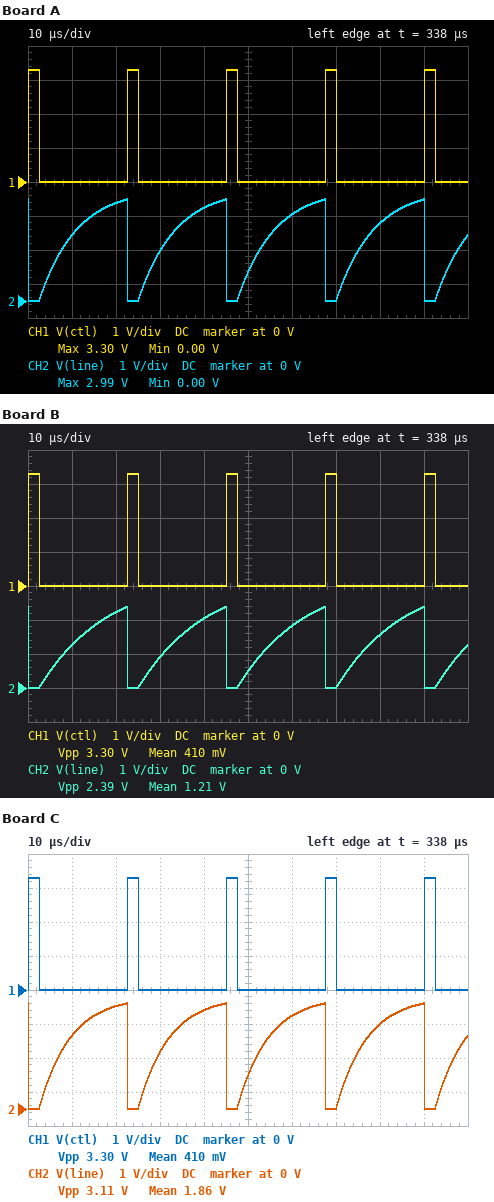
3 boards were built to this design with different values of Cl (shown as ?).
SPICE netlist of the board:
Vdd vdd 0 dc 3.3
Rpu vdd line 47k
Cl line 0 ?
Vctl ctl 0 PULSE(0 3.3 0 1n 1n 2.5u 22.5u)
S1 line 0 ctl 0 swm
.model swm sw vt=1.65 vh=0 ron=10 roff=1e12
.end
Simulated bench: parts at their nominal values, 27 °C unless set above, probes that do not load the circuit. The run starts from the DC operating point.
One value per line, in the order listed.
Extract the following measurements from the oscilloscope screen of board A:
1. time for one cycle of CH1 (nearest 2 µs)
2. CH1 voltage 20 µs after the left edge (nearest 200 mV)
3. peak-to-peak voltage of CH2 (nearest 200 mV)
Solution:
22 µs
0 V
3.0 V
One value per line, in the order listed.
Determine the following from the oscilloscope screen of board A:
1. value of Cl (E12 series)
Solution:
180 pF
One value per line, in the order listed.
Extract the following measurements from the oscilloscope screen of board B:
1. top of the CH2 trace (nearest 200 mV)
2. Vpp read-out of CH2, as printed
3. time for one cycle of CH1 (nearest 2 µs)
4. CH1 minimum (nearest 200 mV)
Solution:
2.4 V
2.39 V
22 µs
0 V
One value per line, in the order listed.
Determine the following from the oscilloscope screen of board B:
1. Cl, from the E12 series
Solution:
330 pF
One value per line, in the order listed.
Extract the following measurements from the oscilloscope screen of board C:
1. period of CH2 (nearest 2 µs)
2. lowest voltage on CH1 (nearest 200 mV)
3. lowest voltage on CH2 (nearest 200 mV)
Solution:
22 µs
0 V
0 V
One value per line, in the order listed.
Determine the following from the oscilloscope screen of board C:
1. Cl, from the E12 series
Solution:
150 pF
